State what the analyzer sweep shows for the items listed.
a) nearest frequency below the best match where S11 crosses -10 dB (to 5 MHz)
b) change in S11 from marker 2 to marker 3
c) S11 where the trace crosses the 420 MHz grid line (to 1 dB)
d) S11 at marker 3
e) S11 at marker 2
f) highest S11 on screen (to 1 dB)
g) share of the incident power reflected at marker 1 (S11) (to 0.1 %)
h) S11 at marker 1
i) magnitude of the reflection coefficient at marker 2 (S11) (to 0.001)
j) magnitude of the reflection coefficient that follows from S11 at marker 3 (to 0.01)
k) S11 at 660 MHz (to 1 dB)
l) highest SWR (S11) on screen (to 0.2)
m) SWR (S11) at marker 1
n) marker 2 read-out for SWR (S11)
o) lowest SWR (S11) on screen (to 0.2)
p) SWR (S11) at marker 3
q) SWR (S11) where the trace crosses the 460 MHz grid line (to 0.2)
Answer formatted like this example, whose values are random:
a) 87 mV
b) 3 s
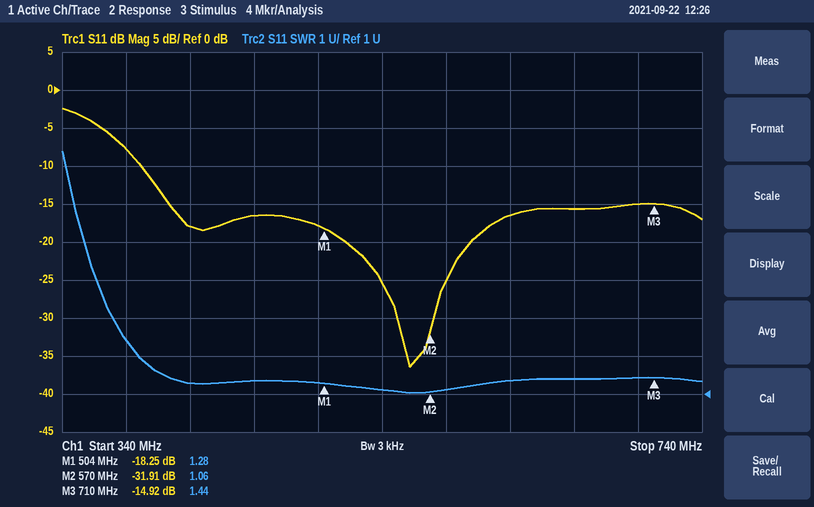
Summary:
a) 390 MHz
b) 16.99 dB
c) -18 dB
d) -14.92 dB
e) -31.91 dB
f) -2 dB
g) 1.5 %
h) -18.25 dB
i) 0.025
j) 0.18
k) -16 dB
l) 7.4
m) 1.28
n) 1.06
o) 1.0
p) 1.44
q) 1.4
